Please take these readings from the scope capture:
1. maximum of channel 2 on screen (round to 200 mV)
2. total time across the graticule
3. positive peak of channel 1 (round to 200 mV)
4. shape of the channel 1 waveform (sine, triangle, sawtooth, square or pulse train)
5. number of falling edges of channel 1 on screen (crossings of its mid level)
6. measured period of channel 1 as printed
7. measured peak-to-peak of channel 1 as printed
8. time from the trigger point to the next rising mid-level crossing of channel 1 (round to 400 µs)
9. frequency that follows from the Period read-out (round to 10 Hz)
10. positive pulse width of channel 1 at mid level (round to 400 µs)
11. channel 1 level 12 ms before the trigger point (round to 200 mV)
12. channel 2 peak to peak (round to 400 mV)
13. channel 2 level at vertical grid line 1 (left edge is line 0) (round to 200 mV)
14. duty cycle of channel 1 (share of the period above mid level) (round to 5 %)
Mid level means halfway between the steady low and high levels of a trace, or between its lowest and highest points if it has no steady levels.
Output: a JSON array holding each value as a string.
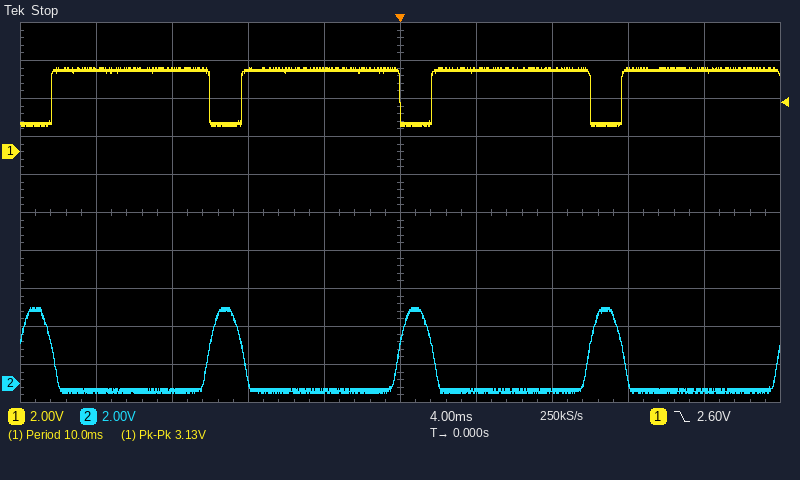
["4.0 V", "40 ms", "4.4 V", "pulse train", "3", "10.0 ms", "3.13 V", "1.6 ms", "100 Hz", "8.4 ms", "4.4 V", "4.4 V", "-400 mV", "85 %"]
